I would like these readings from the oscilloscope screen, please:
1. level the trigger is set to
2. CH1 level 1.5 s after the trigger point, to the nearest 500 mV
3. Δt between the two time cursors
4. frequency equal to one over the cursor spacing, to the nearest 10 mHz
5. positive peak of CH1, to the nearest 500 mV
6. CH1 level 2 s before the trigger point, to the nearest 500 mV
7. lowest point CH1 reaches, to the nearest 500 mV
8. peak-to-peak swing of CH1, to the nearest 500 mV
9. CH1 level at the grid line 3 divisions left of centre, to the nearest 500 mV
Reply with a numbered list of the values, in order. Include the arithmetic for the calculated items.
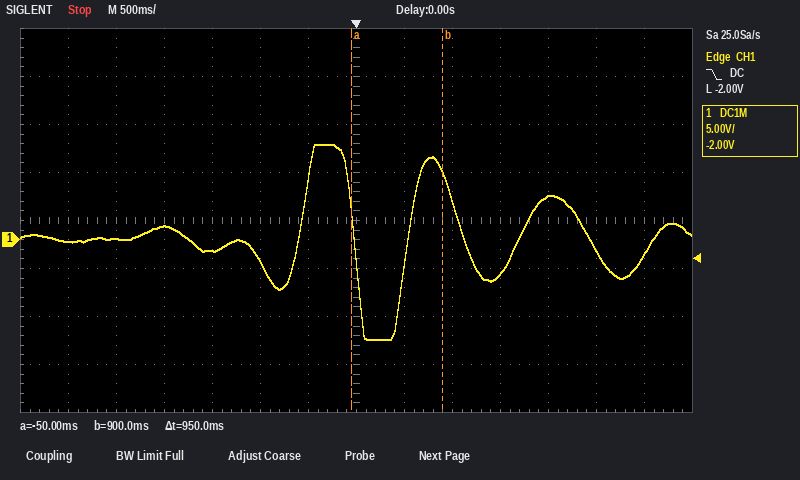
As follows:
1. -2.00 V
2. -3.5 V
3. 950 ms
4. 1 / 950 ms ≈ 1.05 Hz
5. 10.0 V
6. 1.5 V
7. -10.5 V
8. 10.0 V − (-10.5 V) = 20.5 V
9. -1.0 V
